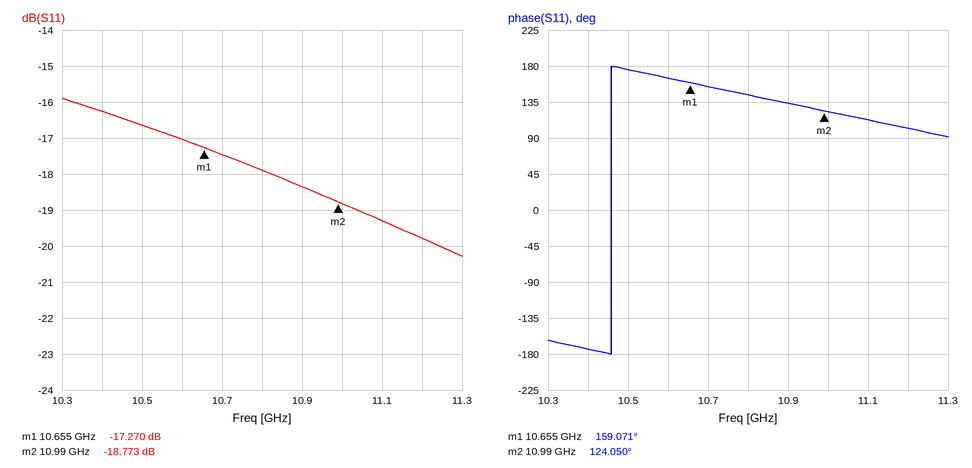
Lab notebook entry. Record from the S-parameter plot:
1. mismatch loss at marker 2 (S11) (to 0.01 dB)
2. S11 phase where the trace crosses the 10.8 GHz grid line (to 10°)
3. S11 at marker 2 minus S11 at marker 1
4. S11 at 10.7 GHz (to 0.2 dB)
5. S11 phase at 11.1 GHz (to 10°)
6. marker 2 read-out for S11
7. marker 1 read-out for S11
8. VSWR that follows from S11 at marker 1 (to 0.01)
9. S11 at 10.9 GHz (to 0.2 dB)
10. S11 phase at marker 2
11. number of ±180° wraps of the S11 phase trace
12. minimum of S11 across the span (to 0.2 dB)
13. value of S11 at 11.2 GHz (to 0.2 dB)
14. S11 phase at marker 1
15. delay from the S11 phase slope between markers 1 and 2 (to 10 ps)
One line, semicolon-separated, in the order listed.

0.06 dB; 140°; -1.503 dB; -17.4 dB; 110°; -18.773 dB; -17.270 dB; 1.32; -18.4 dB; 124.050°; 1; -20.2 dB; -19.8 dB; 159.071°; 290 ps
